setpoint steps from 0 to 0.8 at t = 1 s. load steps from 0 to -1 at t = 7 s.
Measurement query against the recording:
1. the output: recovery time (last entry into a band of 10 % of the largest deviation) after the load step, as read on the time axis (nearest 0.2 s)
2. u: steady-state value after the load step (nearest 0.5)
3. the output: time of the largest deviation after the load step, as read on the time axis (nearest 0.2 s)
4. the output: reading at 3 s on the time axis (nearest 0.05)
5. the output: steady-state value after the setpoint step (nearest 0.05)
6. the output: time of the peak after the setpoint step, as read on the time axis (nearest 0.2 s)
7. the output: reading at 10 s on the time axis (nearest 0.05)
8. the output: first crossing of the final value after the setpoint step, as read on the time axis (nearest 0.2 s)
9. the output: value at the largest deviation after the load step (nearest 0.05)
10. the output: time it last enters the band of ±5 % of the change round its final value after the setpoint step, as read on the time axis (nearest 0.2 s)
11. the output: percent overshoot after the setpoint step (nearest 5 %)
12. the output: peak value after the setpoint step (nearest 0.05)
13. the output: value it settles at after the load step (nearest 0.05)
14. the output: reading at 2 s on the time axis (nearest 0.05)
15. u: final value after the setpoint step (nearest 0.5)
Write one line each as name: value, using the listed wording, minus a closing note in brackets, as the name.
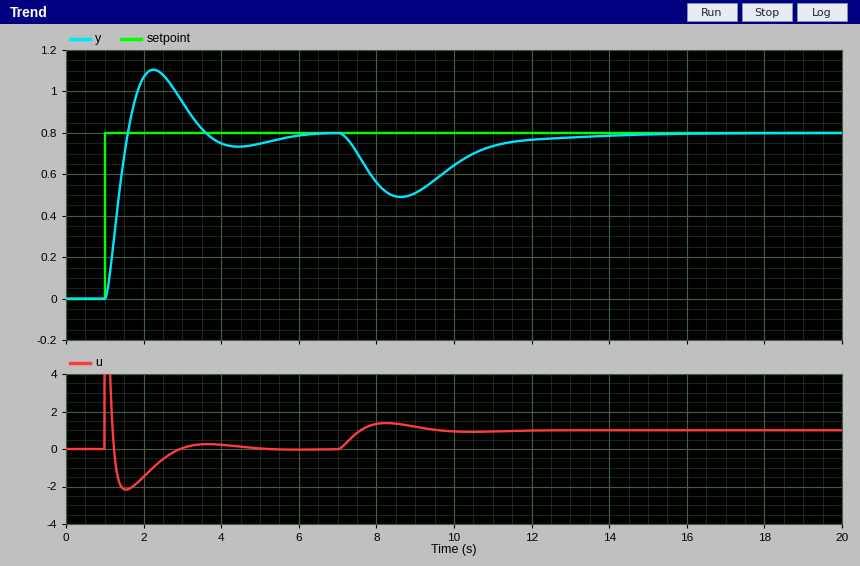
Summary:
the output: recovery time (last entry into a band of 10 % of the largest deviation) after the load step, as read on the time axis: 12.2 s
u: steady-state value after the load step: 1.0
the output: time of the largest deviation after the load step, as read on the time axis: 8.6 s
the output: reading at 3 s on the time axis: 0.95
the output: steady-state value after the setpoint step: 0.80
the output: time of the peak after the setpoint step, as read on the time axis: 2.2 s
the output: reading at 10 s on the time axis: 0.65
the output: first crossing of the final value after the setpoint step, as read on the time axis: 1.6 s
the output: value at the largest deviation after the load step: 0.50
the output: time it last enters the band of ±5 % of the change round its final value after the setpoint step, as read on the time axis: 5.2 s
the output: percent overshoot after the setpoint step: 40 %
the output: peak value after the setpoint step: 1.10
the output: value it settles at after the load step: 0.80
the output: reading at 2 s on the time axis: 1.05
u: final value after the setpoint step: 0.0
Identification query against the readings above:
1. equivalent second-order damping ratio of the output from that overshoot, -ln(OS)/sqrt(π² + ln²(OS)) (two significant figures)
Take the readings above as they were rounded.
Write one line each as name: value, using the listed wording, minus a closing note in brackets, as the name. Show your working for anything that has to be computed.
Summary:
equivalent second-order damping ratio of the output from that overshoot, -ln(OS)/sqrt(π² + ln²(OS)): ln(0.4) = -0.916; 0.916 / sqrt(9.870 + 0.840) = 0.28
